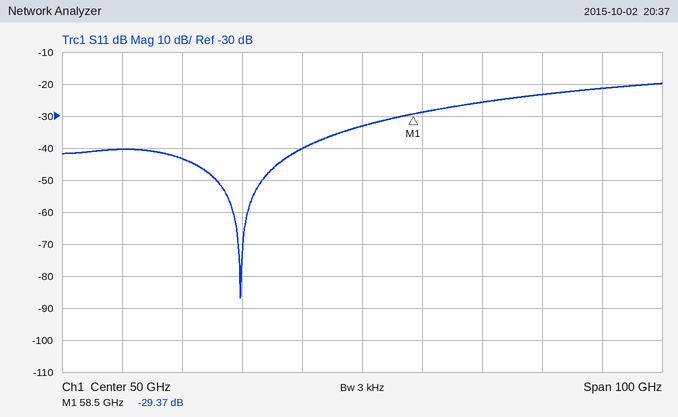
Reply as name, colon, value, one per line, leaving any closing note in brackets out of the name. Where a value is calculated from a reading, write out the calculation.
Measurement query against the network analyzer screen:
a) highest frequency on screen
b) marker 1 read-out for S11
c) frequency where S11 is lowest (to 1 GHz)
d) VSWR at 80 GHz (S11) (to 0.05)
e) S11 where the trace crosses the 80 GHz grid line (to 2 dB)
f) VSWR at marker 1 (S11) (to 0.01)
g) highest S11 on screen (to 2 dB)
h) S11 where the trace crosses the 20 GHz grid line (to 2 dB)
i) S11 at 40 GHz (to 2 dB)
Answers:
highest frequency on screen: 100 GHz
marker 1 read-out for S11: -29.37 dB
frequency where S11 is lowest: 30 GHz
VSWR at 80 GHz (S11): |Γ| = 10^(-24/20) = 0.0631; VSWR = (1 + 0.0631)/(1 − 0.0631) ≈ 1.13, so 1.15 to the nearest 0.05
S11 where the trace crosses the 80 GHz grid line: -24 dB
VSWR at marker 1 (S11): (1 + 0.0340)/(1 − 0.0340) ≈ 1.07
highest S11 on screen: -20 dB
S11 where the trace crosses the 20 GHz grid line: -44 dB
S11 at 40 GHz: -40 dB
